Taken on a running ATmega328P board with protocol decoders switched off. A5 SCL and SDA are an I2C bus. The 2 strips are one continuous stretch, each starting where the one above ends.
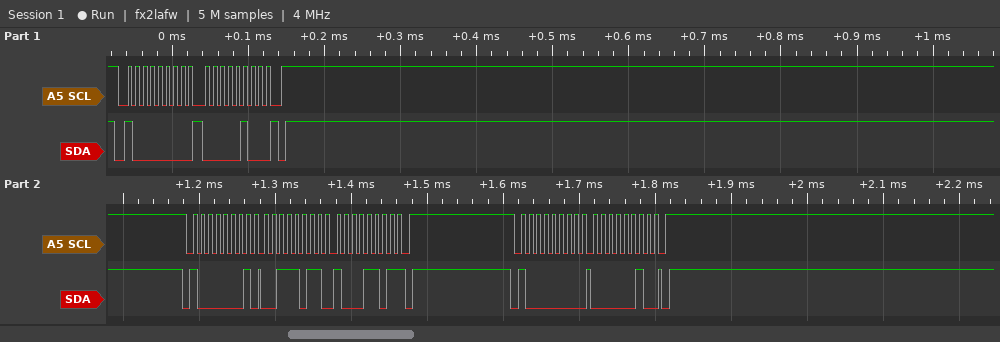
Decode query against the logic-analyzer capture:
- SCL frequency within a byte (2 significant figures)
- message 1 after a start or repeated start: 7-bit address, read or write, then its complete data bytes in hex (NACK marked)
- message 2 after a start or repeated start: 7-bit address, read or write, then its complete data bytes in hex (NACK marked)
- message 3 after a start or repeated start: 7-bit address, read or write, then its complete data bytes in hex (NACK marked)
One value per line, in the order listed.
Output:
100 kHz
0x40 write: 04
0x40 read: 3B 8D NACK
0x40 write: 02
